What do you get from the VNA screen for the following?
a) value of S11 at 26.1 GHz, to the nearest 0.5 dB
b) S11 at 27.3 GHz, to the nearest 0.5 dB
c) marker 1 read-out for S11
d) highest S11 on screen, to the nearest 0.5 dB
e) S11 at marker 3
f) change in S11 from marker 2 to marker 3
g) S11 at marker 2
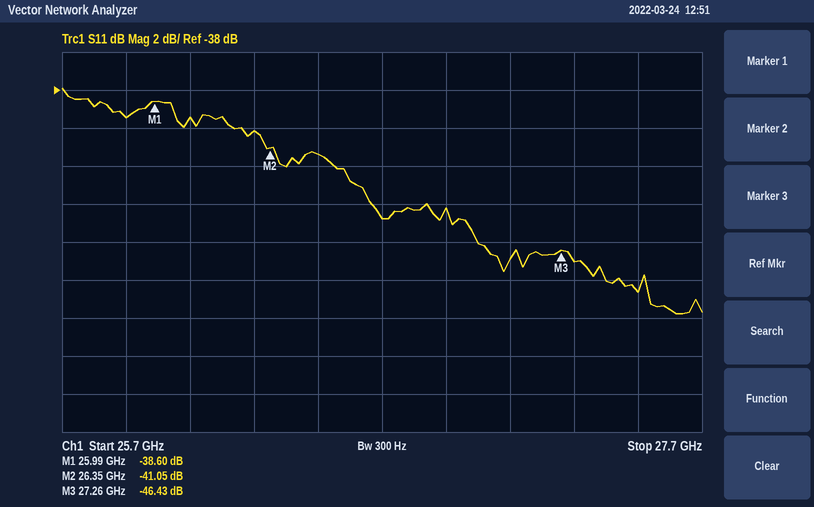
-39.5 dB
-47.0 dB
-38.60 dB
-38.0 dB
-46.43 dB
-5.38 dB
-41.05 dB
